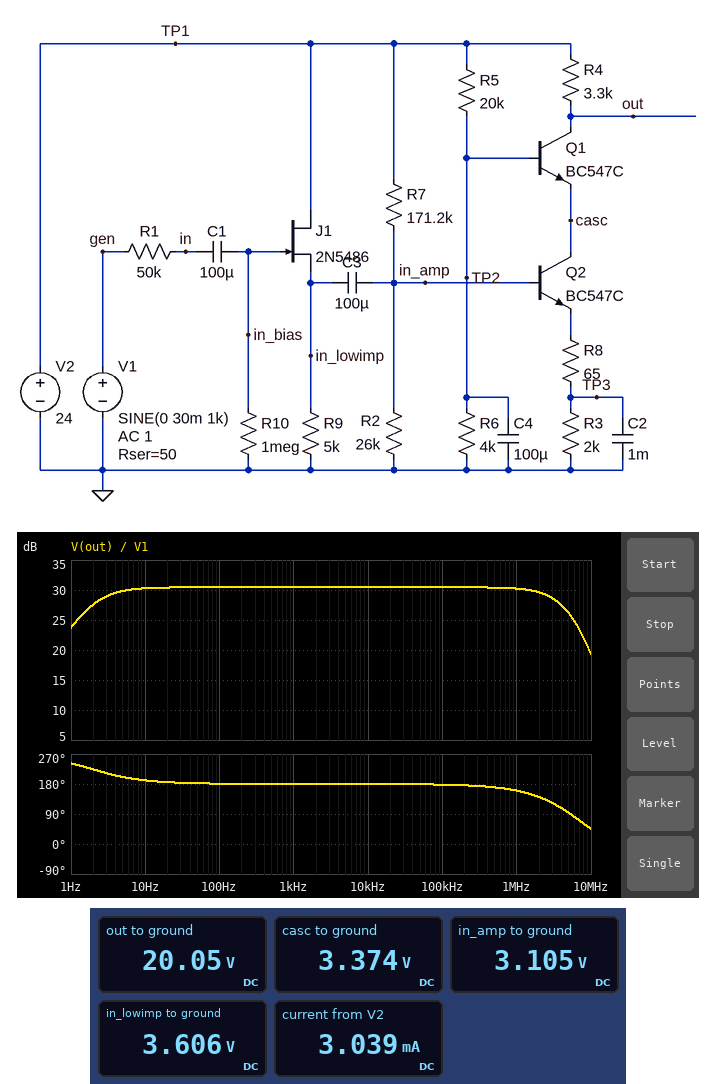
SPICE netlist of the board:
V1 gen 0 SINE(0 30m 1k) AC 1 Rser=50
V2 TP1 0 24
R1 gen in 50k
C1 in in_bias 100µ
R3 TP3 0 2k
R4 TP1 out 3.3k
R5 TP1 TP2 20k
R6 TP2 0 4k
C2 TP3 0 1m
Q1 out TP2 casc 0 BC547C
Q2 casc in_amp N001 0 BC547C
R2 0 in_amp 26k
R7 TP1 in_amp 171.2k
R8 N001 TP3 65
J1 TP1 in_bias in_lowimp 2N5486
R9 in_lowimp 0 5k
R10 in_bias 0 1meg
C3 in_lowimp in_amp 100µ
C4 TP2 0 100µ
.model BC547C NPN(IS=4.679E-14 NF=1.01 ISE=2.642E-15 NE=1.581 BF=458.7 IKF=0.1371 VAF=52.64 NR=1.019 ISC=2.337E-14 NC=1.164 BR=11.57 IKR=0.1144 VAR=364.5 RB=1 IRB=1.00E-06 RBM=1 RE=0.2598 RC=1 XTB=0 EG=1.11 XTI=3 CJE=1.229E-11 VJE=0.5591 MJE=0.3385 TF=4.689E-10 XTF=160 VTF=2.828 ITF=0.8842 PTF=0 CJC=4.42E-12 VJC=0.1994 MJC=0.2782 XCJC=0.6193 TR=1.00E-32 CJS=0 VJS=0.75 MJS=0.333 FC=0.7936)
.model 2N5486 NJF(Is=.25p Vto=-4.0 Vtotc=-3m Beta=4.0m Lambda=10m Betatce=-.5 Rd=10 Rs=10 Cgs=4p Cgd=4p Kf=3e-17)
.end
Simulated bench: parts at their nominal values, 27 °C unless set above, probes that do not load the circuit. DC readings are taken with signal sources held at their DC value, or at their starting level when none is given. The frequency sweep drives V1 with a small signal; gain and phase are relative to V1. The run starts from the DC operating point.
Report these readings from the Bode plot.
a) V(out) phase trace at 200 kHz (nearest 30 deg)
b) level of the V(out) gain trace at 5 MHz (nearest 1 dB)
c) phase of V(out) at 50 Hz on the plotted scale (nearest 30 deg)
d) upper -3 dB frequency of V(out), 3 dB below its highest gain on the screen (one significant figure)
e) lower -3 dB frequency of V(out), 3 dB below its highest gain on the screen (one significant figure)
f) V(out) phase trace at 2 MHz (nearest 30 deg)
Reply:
180 deg
26 dB
180 deg
4 MHz
2 Hz
150 deg
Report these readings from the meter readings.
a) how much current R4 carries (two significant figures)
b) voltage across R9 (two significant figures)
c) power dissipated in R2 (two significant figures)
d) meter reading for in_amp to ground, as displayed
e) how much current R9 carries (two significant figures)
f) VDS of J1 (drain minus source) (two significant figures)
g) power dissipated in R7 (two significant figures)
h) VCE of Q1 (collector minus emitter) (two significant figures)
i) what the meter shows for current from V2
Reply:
1.2 mA
3.6 V
370 µW
3.105 V
720 µA
20 V
2.6 mW
17 V
3.039 mA
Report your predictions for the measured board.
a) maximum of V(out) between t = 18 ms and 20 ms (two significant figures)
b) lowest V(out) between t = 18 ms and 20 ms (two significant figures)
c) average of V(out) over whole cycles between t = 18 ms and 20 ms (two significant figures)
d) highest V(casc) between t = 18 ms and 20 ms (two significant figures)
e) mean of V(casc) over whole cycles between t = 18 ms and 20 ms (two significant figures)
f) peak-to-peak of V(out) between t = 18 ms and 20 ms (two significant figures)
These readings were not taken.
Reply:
21 V
19 V
20 V
3.4 V
3.4 V
2.0 V
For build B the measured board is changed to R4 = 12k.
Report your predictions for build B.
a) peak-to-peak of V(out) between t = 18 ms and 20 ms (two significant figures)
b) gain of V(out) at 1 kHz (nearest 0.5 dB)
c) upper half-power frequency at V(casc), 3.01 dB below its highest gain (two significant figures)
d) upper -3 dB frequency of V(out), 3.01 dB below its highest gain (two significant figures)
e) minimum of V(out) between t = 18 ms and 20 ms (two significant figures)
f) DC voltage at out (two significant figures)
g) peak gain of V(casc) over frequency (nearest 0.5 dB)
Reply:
7.2 V
41.5 dB
3.8 MHz
3.4 MHz
5.9 V
9.7 V
-11.0 dB
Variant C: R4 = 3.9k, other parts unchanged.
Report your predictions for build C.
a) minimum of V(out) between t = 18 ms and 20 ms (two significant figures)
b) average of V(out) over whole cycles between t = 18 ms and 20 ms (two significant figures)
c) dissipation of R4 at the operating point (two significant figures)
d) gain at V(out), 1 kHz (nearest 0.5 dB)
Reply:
18 V
19 V
5.6 mW
32.0 dB
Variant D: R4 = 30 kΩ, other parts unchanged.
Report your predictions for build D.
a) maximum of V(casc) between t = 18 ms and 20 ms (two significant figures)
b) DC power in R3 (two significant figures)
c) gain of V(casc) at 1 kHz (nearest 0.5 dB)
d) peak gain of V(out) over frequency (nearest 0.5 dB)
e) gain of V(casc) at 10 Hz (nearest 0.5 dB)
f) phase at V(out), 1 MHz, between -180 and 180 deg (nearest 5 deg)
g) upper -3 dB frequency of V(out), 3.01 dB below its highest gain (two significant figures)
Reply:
2.3 V
2.3 mW
-7.0 dB
4.5 dB
0.5 dB
150 deg
9.1 Hz
